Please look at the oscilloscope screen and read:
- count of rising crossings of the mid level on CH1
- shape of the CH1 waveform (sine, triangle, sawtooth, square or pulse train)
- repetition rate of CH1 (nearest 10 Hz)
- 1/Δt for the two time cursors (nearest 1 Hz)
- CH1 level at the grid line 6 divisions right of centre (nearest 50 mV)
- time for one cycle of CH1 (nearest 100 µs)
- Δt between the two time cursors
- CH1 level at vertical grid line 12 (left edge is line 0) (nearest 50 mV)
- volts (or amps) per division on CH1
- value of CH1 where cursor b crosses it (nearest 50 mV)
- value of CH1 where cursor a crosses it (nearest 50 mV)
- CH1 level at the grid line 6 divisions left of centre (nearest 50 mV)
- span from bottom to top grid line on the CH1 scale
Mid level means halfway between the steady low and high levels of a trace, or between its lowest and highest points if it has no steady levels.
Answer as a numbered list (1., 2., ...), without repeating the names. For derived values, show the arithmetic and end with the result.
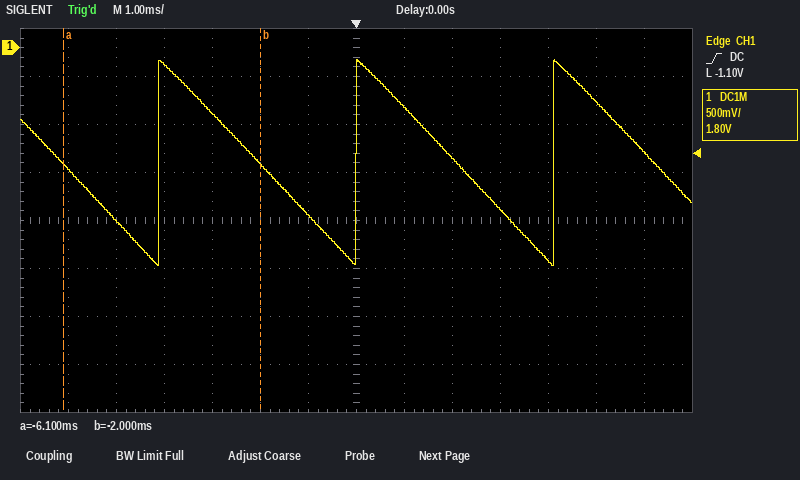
1. 3
2. sawtooth
3. 1 / 4.1 ms ≈ 244 Hz, so 240 Hz to the nearest 10 Hz
4. 1 / 4.1 ms ≈ 244 Hz
5. -1.10 V
6. 4.1 ms
7. -2 ms − (-6.1 ms) = 4.1 ms
8. -550 mV
9. 500 mV
10. -1.20 V
11. -1.20 V
12. -1.25 V
13. 4 V
